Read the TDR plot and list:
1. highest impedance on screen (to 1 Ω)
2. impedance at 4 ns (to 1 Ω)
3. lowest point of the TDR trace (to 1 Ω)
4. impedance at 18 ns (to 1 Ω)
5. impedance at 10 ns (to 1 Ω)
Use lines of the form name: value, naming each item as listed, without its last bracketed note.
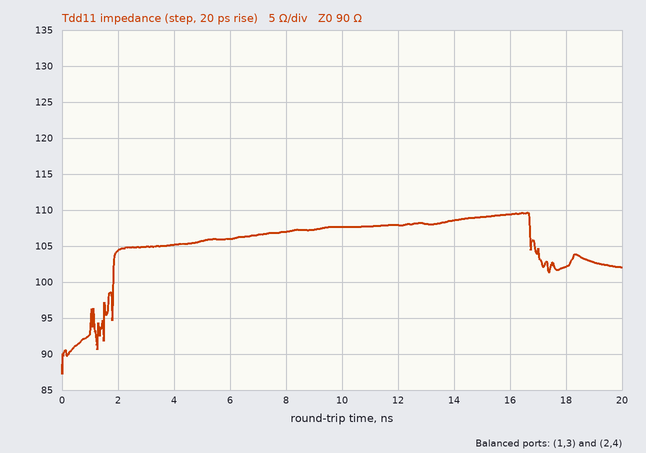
highest impedance on screen: 110 Ω
impedance at 4 ns: 105 Ω
lowest point of the TDR trace: 87 Ω
impedance at 18 ns: 102 Ω
impedance at 10 ns: 108 Ω
